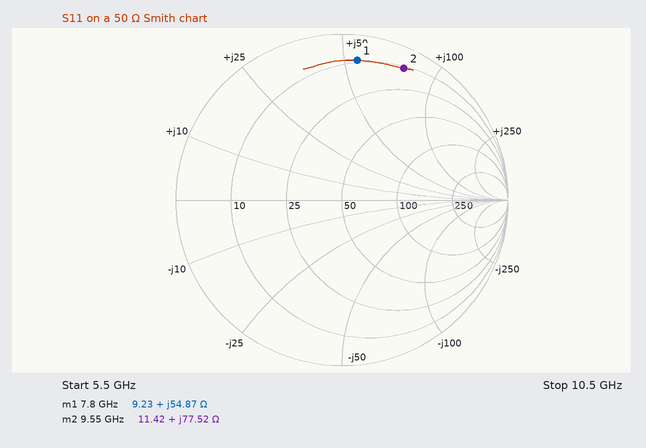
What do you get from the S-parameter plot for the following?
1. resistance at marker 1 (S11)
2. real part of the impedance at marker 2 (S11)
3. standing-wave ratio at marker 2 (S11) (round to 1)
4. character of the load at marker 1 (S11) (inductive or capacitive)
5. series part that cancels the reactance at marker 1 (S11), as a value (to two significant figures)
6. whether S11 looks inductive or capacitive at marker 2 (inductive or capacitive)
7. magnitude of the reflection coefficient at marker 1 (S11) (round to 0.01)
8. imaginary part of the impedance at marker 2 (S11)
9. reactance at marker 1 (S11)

9.23 Ω
11.42 Ω
15
inductive
370 fF
inductive
0.85
+77.52 Ω
+54.87 Ω
